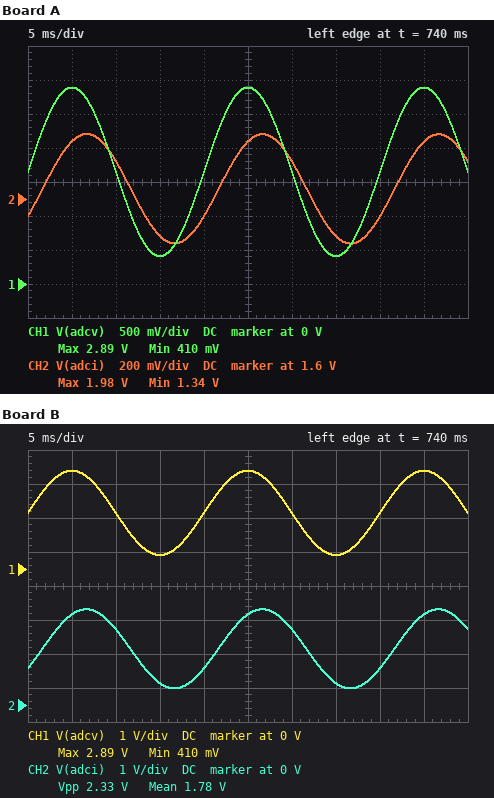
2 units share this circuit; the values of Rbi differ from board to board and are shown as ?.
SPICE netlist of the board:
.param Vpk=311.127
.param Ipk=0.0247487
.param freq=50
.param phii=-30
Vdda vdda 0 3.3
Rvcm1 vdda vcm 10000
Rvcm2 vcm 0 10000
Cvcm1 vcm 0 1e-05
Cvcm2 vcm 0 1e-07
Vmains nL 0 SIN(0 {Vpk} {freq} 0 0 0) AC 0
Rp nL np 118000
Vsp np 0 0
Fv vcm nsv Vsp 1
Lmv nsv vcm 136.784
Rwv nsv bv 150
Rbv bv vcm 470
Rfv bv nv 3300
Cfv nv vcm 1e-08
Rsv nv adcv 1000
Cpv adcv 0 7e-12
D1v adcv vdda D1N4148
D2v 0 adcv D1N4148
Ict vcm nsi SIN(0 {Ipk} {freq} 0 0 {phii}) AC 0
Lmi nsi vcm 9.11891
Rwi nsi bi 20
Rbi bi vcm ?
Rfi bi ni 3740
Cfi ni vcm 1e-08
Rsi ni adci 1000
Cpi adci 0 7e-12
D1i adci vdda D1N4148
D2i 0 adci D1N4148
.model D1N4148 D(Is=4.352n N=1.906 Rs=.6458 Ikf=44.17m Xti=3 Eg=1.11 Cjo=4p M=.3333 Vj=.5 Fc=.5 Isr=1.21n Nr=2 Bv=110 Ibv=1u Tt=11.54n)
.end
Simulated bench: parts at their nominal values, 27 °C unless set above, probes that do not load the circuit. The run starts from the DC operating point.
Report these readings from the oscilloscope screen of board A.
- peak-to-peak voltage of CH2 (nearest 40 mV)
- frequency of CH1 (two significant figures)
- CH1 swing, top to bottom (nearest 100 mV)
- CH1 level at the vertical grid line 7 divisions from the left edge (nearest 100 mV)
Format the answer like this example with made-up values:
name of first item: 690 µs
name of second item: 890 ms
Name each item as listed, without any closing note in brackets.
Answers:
peak-to-peak voltage of CH2: 640 mV
frequency of CH1: 50 Hz
CH1 swing, top to bottom: 2.5 V
CH1 level at the vertical grid line 7 divisions from the left edge: 400 mV
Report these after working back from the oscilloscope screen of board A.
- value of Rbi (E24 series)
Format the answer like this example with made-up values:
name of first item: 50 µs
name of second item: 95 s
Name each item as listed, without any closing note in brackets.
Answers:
value of Rbi: 13 Ω
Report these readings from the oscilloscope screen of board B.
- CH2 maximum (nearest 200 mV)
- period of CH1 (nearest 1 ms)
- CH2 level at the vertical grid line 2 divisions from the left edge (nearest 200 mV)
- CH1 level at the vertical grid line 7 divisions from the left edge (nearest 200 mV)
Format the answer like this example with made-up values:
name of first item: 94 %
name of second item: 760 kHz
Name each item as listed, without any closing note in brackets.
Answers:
CH2 maximum: 2.8 V
period of CH1: 20 ms
CH2 level at the vertical grid line 2 divisions from the left edge: 2.2 V
CH1 level at the vertical grid line 7 divisions from the left edge: 400 mV
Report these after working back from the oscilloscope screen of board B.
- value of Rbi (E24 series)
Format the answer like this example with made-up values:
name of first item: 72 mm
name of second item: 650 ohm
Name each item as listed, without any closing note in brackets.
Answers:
value of Rbi: 47 Ω
